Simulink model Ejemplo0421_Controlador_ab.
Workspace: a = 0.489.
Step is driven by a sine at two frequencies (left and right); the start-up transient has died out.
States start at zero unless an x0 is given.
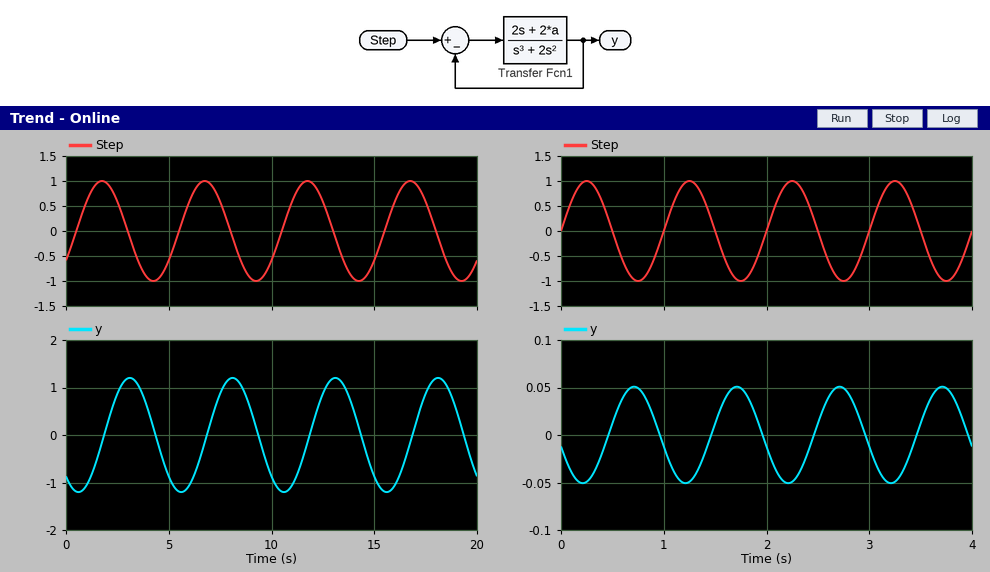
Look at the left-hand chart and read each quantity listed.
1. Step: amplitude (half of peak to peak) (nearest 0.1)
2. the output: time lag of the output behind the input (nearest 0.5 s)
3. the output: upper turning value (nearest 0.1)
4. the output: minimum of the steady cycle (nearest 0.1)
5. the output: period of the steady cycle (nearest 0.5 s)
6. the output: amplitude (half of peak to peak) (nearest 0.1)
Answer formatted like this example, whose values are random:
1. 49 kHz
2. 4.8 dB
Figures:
1. 1.0
2. 1.5 s
3. 1.2
4. -1.2
5. 5.0 s
6. 1.2
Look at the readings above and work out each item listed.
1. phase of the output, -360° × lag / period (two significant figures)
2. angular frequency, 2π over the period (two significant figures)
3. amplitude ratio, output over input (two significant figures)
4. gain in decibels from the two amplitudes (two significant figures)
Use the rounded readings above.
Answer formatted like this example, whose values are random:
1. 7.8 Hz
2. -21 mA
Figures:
1. -110°
2. 1.3 rad/s
3. 1.2
4. 1.6 dB
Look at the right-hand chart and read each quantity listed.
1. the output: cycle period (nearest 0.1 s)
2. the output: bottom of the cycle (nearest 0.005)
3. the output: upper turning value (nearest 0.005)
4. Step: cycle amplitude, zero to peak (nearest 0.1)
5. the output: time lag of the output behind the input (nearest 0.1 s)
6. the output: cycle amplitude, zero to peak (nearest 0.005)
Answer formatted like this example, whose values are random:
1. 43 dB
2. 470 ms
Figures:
1. 1.0 s
2. -0.050
3. 0.050
4. 1.0
5. 0.5 s
6. 0.050
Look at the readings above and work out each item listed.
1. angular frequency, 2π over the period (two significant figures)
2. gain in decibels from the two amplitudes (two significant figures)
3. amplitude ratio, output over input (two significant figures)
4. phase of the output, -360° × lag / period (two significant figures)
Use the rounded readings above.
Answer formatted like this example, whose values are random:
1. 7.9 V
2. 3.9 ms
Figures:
1. 6.3 rad/s
2. -26 dB
3. 0.050
4. -180°
